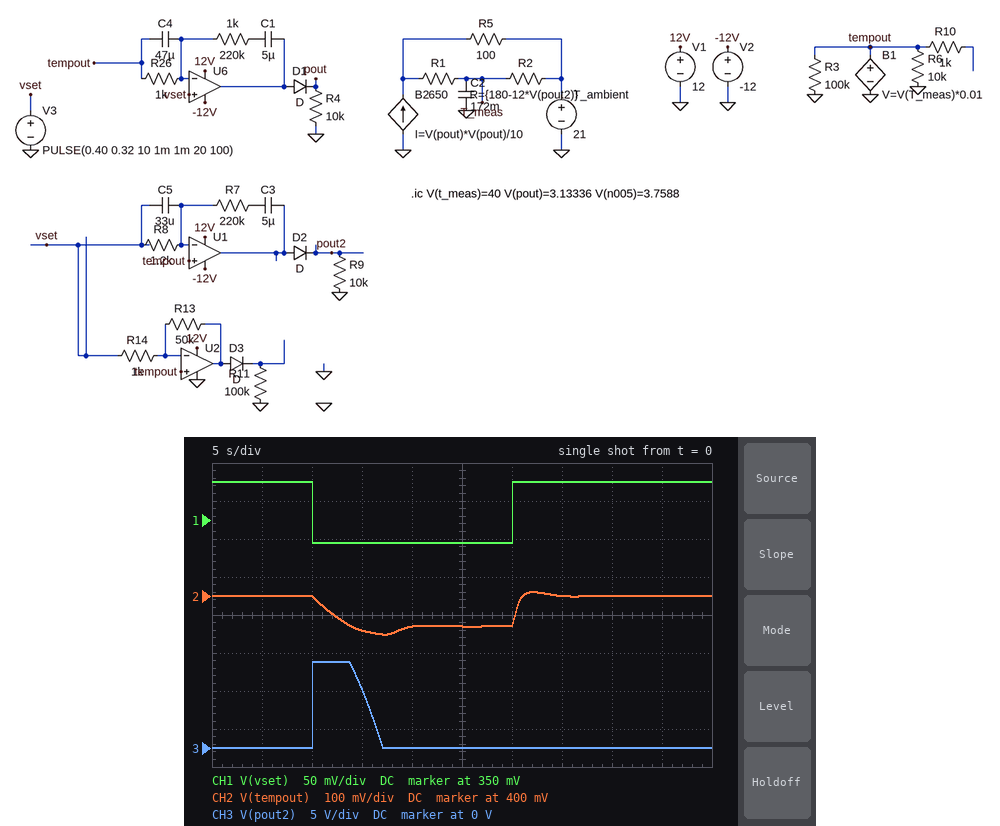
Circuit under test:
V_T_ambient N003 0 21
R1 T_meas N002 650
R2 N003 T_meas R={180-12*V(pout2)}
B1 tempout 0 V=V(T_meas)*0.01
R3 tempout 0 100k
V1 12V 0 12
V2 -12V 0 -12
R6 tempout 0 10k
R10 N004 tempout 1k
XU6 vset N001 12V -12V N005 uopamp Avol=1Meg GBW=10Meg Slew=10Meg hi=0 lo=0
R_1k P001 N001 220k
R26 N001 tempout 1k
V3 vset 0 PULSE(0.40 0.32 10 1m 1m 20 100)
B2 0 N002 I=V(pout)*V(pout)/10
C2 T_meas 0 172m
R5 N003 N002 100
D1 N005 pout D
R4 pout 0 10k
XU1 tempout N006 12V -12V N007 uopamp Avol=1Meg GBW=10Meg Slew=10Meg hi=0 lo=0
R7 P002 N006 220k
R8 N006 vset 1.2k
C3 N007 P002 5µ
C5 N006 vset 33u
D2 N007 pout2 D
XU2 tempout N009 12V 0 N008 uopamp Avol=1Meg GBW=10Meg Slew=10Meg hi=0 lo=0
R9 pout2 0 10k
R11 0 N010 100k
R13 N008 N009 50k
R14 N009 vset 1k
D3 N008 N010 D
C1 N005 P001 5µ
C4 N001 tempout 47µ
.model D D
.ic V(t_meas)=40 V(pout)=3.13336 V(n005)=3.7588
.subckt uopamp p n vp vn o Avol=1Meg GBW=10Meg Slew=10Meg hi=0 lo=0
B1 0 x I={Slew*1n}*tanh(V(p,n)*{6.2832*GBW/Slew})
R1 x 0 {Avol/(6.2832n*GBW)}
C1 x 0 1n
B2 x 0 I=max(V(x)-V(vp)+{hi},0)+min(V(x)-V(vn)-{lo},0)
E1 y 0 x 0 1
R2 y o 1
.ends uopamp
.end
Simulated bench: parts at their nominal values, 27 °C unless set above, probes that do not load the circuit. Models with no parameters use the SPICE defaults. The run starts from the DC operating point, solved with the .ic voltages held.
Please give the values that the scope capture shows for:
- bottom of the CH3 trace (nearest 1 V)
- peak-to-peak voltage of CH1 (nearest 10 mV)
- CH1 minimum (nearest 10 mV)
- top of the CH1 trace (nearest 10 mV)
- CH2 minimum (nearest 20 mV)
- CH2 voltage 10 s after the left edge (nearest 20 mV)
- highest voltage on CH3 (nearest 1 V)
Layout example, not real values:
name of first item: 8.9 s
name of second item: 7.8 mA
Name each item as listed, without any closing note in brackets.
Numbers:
bottom of the CH3 trace: 0 V
peak-to-peak voltage of CH1: 80 mV
CH1 minimum: 320 mV
top of the CH1 trace: 400 mV
CH2 minimum: 300 mV
CH2 voltage 10 s after the left edge: 400 mV
highest voltage on CH3: 11 V
